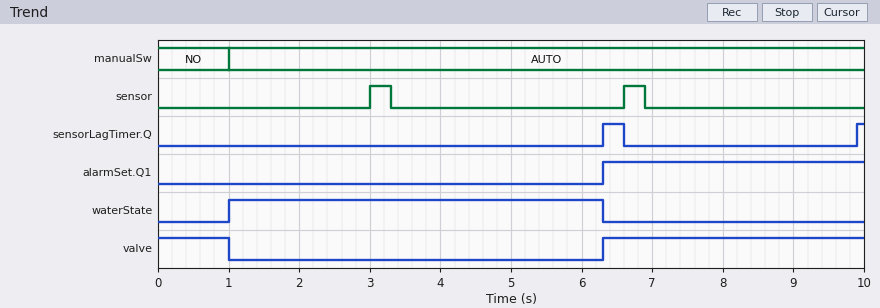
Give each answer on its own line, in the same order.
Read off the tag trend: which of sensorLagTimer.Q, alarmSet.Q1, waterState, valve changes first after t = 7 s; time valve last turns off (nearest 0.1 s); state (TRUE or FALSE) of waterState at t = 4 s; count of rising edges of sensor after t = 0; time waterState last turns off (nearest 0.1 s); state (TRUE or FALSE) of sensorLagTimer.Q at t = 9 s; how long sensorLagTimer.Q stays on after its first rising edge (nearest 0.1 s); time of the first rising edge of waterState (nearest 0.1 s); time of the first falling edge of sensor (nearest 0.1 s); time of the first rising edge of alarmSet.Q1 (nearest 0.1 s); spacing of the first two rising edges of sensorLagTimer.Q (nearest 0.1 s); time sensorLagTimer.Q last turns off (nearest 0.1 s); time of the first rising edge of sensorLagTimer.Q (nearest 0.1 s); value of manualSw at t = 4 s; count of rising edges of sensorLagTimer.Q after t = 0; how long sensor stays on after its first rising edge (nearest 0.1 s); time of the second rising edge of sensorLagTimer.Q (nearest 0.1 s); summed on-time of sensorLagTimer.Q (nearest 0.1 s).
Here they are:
sensorLagTimer.Q
1.0 s
TRUE
2
6.3 s
FALSE
0.3 s
1.0 s
3.3 s
6.3 s
3.6 s
6.6 s
6.3 s
AUTO
2
0.3 s
9.9 s
0.4 s
